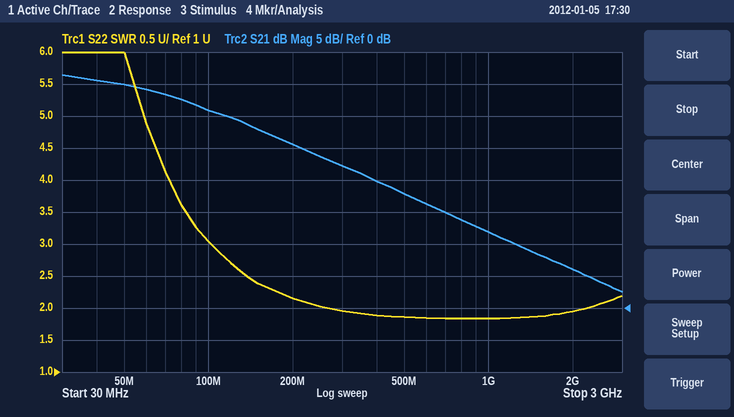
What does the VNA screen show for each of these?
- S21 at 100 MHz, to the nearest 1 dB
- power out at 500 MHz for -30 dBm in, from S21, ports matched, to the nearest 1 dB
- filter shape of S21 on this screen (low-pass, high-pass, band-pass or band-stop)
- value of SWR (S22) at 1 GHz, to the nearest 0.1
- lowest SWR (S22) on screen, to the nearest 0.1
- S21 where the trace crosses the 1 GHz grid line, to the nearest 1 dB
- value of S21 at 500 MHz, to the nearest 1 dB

31 dB
-12 dBm
low-pass
1.8
1.8
12 dB
18 dB
